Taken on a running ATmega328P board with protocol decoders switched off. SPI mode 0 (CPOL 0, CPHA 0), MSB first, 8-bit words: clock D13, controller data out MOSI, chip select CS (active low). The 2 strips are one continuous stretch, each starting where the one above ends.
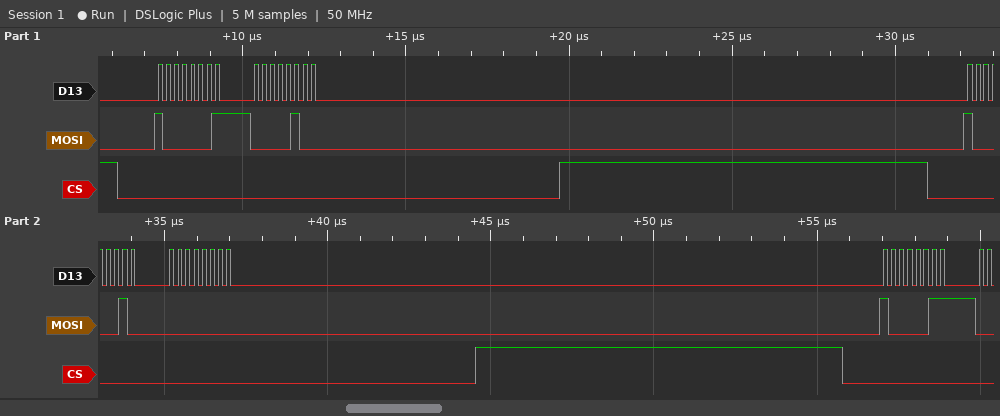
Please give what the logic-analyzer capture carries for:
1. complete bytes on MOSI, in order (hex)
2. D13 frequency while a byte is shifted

0x81 0x04 0x82 0x00 0x83
4 MHz
